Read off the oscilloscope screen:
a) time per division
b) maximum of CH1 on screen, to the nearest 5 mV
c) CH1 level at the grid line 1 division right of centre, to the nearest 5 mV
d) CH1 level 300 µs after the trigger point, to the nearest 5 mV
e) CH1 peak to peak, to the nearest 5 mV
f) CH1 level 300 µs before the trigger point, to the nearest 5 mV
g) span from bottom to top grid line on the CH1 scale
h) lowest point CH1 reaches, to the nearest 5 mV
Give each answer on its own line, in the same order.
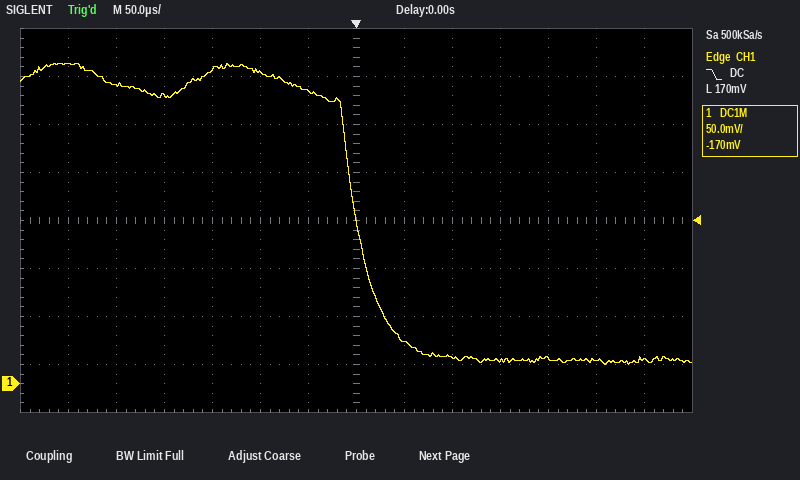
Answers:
50 µs
335 mV
45 mV
25 mV
315 mV
335 mV
400 mV
20 mV
